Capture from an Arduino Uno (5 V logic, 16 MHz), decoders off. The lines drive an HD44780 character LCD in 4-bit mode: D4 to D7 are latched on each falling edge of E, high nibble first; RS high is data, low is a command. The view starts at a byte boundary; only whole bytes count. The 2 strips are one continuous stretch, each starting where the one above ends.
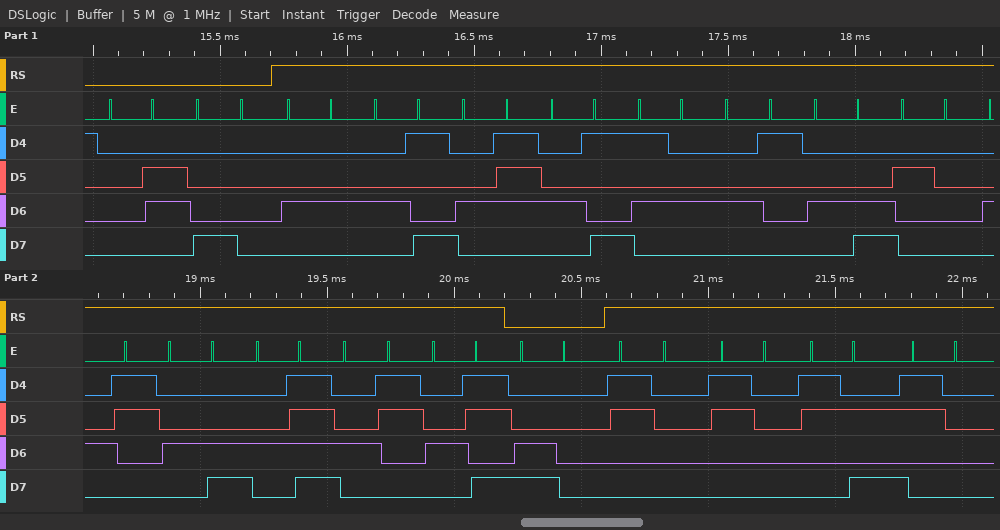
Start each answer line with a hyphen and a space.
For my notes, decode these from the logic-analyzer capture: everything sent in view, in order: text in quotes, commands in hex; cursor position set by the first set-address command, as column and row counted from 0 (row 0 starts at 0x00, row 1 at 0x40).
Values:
- 0x06 0x80 "DIGITAL CLOCK" 0xC0 "00:0"
- column 0, row 0
